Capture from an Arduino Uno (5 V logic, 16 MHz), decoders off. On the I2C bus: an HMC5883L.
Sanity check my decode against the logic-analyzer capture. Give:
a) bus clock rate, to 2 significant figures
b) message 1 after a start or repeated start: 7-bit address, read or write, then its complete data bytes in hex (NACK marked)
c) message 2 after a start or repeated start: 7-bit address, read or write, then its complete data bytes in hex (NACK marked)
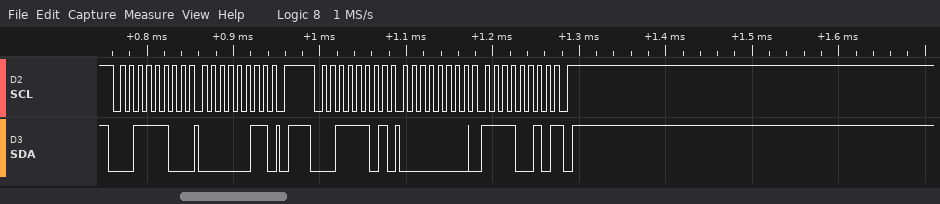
100 kHz
0x1E write: 03
0x1E read: 00 F2 NACK
